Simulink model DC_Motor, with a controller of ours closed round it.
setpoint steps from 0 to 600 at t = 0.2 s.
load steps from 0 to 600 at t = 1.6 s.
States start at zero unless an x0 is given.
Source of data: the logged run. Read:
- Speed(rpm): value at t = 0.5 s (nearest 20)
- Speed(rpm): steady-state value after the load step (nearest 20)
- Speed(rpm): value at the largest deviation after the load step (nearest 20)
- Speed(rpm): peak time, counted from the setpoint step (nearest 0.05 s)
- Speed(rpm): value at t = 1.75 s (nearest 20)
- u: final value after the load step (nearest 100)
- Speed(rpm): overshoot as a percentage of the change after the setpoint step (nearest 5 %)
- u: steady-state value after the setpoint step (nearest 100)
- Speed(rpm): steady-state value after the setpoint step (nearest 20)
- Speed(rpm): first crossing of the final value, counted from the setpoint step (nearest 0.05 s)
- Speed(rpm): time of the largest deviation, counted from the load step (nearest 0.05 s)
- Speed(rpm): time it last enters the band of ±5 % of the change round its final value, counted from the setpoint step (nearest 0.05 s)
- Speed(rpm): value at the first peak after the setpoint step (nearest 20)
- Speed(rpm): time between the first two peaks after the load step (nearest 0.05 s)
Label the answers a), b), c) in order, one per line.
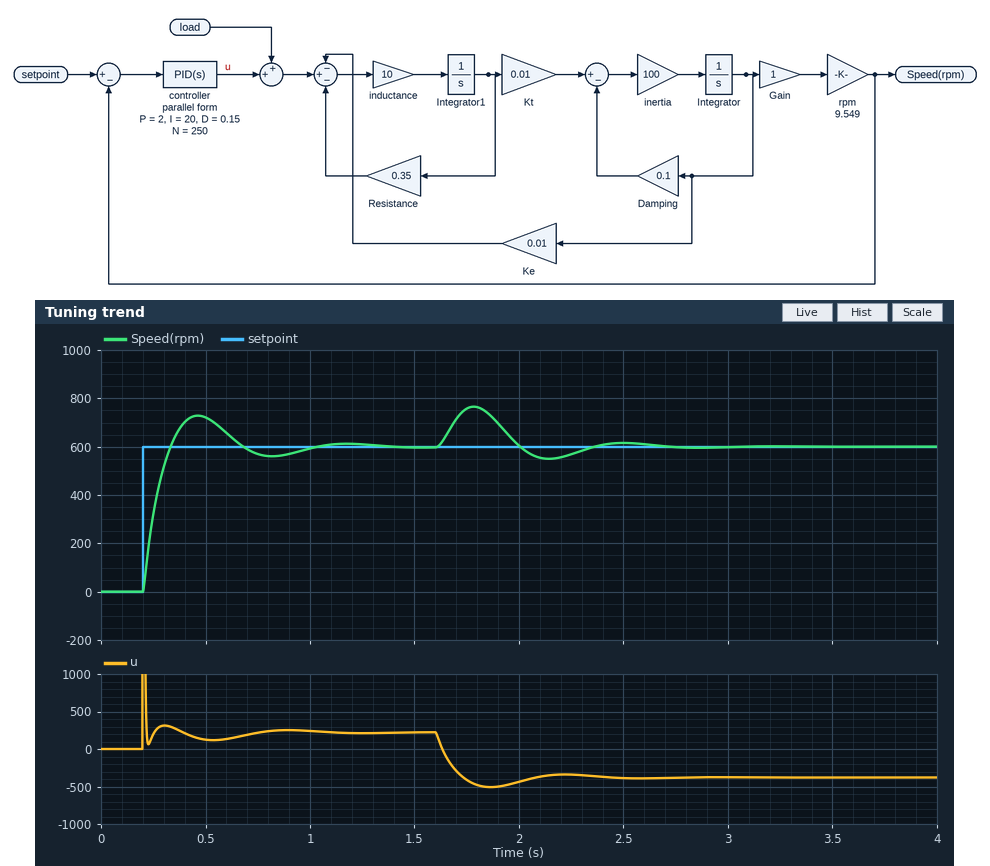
a) 720
b) 600
c) 760
d) 0.25 s
e) 760
f) -400
g) 20 %
h) 200
i) 600
j) 0.15 s
k) 0.20 s
l) 0.70 s
m) 720
n) 0.70 s
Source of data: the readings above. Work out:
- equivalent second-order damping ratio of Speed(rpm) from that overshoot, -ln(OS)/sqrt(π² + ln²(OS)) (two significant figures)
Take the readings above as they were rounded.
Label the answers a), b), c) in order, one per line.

a) 0.46
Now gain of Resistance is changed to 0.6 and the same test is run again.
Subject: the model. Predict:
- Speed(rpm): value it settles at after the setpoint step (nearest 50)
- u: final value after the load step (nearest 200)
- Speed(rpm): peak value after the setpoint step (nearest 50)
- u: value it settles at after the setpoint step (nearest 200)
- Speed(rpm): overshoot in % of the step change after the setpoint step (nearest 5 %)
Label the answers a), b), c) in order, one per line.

a) 600
b) -200
c) 700
d) 400
e) 15 %
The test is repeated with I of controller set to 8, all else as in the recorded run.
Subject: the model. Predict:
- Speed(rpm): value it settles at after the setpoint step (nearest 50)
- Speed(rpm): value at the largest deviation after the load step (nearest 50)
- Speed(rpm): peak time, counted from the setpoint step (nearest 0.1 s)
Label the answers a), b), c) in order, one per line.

a) 600
b) 800
c) 0.4 s
